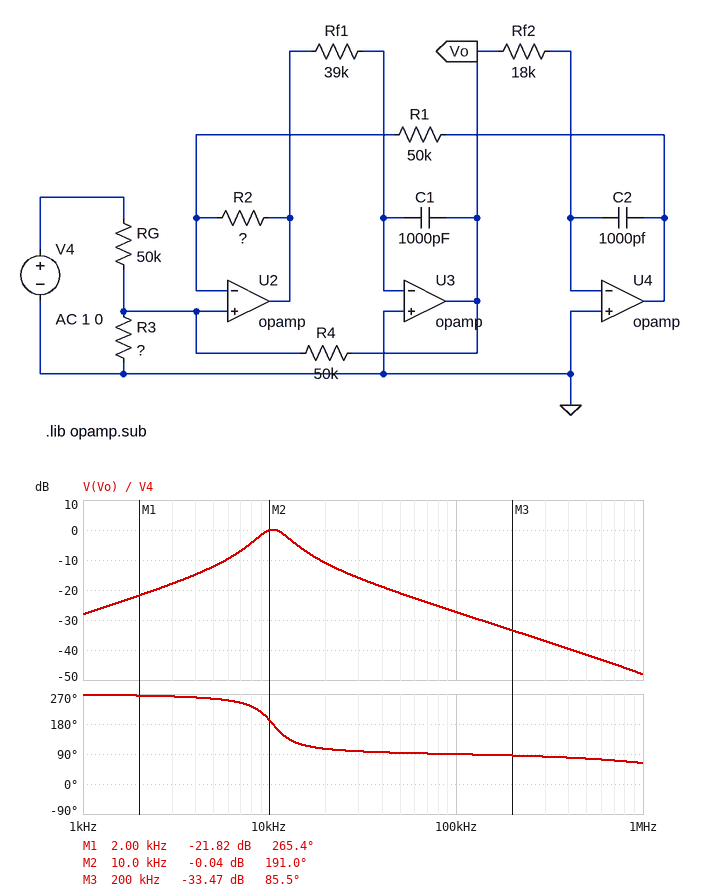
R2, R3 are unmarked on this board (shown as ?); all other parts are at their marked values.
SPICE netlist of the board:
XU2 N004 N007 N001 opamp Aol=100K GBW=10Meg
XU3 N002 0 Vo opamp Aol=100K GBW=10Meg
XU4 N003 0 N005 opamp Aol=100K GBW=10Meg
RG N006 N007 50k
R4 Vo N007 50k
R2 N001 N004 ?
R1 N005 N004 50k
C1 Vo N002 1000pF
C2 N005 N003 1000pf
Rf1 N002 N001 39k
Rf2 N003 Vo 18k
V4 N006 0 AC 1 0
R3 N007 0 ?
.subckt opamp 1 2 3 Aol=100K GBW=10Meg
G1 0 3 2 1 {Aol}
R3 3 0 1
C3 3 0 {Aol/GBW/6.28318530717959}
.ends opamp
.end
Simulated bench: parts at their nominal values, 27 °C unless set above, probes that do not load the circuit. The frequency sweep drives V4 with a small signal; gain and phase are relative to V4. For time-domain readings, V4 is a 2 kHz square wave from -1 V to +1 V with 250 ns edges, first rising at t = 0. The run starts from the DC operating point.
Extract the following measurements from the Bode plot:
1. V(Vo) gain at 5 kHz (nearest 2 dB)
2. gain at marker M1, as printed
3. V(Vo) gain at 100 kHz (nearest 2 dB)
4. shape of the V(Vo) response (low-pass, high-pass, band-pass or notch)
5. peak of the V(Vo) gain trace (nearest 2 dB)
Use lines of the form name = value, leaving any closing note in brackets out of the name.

V(Vo) gain at 5 kHz = -12 dB
gain at marker M1, as printed = -21.82 dB
V(Vo) gain at 100 kHz = -28 dB
shape of the V(Vo) response = band-pass
peak of the V(Vo) gain trace = 0 dB
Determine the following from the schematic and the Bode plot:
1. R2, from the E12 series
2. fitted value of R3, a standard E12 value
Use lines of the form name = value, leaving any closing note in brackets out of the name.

R2, from the E12 series = 150 kΩ
fitted value of R3, a standard E12 value = 27 kΩ
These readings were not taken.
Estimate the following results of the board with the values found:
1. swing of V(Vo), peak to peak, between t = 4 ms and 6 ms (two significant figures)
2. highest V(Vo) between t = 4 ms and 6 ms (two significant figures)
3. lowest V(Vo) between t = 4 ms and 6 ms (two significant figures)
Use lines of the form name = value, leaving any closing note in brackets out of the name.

swing of V(Vo), peak to peak, between t = 4 ms and 6 ms = 1.3 V
highest V(Vo) between t = 4 ms and 6 ms = 640 mV
lowest V(Vo) between t = 4 ms and 6 ms = -640 mV
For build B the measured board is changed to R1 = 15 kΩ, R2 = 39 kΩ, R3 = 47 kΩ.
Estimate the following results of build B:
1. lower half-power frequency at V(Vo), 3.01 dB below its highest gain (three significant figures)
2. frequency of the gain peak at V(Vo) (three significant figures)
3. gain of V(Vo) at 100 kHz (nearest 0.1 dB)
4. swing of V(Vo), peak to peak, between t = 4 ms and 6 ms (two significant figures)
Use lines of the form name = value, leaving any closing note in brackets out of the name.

lower half-power frequency at V(Vo), 3.01 dB below its highest gain = 7.60 kHz
frequency of the gain peak at V(Vo) = 9.69 kHz
gain of V(Vo) at 100 kHz = -26.3 dB
swing of V(Vo), peak to peak, between t = 4 ms and 6 ms = 1.4 V
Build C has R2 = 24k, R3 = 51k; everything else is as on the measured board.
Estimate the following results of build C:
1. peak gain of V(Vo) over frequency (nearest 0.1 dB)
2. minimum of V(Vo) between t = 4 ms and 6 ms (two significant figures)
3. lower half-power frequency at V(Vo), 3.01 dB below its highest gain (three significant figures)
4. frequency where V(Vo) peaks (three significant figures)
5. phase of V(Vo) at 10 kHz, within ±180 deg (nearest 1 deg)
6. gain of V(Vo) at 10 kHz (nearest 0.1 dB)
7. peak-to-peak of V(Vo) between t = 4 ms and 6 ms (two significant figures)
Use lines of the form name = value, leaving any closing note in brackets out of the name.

peak gain of V(Vo) over frequency = 0 dB
minimum of V(Vo) between t = 4 ms and 6 ms = -580 mV
lower half-power frequency at V(Vo), 3.01 dB below its highest gain = 3.27 kHz
frequency where V(Vo) peaks = 4.16 kHz
phase of V(Vo) at 10 kHz, within ±180 deg = 104 deg
gain of V(Vo) at 10 kHz = -12.5 dB
peak-to-peak of V(Vo) between t = 4 ms and 6 ms = 1.2 V
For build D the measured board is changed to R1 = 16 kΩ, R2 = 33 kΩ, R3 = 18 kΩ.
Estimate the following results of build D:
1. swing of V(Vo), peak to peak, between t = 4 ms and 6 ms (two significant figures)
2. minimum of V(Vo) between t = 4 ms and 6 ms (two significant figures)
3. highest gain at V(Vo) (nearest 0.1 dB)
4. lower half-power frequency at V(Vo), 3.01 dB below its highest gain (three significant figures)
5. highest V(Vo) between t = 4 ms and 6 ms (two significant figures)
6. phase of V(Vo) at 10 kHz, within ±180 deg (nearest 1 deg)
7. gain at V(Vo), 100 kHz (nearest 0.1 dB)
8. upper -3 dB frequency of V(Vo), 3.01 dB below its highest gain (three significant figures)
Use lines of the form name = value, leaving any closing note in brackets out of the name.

swing of V(Vo), peak to peak, between t = 4 ms and 6 ms = 880 mV
minimum of V(Vo) between t = 4 ms and 6 ms = -440 mV
highest gain at V(Vo) = 0.1 dB
lower half-power frequency at V(Vo), 3.01 dB below its highest gain = 7.43 kHz
highest V(Vo) between t = 4 ms and 6 ms = 440 mV
phase of V(Vo) at 10 kHz, within ±180 deg = 135 deg
gain at V(Vo), 100 kHz = -31.6 dB
upper -3 dB frequency of V(Vo), 3.01 dB below its highest gain = 10.0 kHz
